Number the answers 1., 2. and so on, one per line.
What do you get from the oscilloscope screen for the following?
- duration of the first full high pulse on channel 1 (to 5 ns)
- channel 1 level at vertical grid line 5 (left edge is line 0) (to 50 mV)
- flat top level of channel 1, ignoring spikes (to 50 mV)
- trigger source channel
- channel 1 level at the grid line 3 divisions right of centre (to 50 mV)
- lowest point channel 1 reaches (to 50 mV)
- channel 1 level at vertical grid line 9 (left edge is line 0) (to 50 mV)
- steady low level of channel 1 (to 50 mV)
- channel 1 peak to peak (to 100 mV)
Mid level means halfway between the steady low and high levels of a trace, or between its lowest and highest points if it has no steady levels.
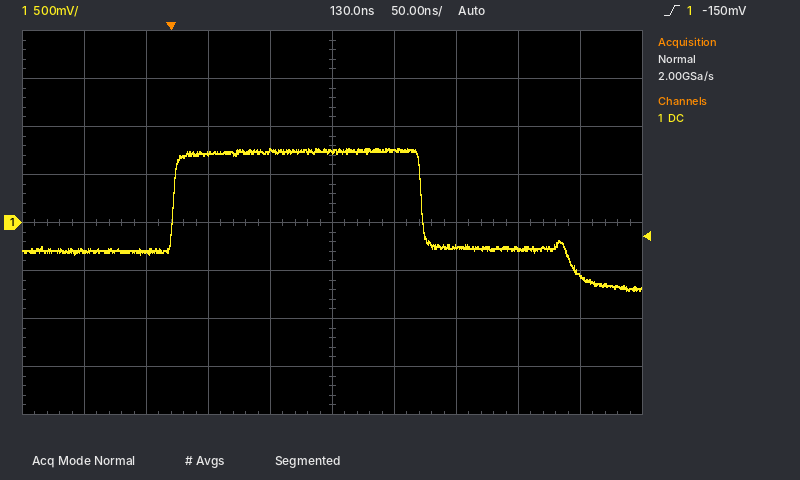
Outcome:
1. 200 ns
2. 750 mV
3. 750 mV
4. channel 1
5. -250 mV
6. -700 mV
7. -550 mV
8. -300 mV
9. 1.50 V
